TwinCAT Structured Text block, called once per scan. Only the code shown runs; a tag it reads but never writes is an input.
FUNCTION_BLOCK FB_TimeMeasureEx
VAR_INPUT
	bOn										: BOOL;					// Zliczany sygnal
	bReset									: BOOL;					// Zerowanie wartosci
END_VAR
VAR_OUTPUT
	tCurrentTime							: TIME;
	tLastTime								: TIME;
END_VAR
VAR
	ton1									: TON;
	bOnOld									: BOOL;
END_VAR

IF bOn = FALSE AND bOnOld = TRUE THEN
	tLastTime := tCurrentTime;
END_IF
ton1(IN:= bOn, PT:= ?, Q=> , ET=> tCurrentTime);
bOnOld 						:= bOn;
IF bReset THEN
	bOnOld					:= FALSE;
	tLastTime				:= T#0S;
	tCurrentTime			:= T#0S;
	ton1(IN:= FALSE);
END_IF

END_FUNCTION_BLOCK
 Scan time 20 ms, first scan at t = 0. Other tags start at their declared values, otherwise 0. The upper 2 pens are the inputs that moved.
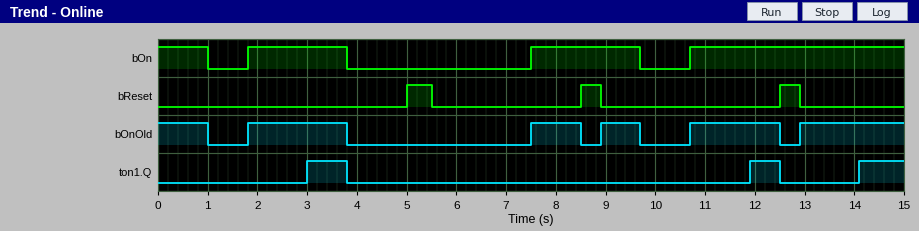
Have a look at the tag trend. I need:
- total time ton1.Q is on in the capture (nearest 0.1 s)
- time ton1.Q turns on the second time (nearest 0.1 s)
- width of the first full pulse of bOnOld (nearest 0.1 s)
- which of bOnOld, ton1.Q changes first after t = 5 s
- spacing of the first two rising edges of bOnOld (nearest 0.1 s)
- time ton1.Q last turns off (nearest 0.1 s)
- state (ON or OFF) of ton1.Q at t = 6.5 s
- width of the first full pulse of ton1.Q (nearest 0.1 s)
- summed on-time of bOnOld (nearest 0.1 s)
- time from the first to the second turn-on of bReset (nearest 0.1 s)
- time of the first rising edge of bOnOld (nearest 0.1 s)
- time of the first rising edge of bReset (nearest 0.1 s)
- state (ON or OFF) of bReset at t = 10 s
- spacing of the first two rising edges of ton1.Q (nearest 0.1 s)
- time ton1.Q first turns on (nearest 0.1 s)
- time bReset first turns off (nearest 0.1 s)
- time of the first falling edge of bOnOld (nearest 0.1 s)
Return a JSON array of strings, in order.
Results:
["2.3 s", "11.9 s", "2.0 s", "bOnOld", "5.7 s", "12.5 s", "OFF", "0.8 s", "8.7 s", "3.5 s", "1.8 s", "5.0 s", "OFF", "8.9 s", "3.0 s", "5.5 s", "1.0 s"]
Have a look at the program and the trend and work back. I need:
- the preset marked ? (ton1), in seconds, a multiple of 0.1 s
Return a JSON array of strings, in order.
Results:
["1.2 s"]
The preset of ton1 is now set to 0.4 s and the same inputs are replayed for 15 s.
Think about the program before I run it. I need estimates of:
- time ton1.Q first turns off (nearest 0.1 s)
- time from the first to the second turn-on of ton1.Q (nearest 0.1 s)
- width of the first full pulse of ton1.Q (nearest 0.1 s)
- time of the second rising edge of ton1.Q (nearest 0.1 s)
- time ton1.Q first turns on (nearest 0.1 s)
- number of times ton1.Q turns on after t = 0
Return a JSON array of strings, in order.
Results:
["1.0 s", "1.8 s", "0.6 s", "2.2 s", "0.4 s", "6"]
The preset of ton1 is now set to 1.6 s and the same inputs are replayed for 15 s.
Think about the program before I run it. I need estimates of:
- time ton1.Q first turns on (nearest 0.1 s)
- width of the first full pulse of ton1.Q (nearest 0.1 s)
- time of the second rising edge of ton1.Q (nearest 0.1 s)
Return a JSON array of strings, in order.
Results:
["3.4 s", "0.4 s", "12.3 s"]
